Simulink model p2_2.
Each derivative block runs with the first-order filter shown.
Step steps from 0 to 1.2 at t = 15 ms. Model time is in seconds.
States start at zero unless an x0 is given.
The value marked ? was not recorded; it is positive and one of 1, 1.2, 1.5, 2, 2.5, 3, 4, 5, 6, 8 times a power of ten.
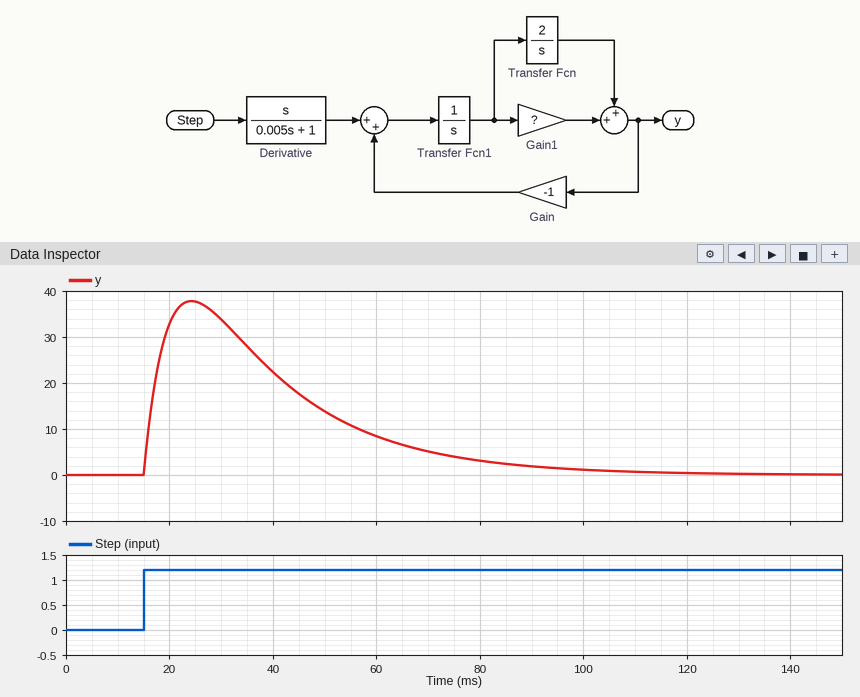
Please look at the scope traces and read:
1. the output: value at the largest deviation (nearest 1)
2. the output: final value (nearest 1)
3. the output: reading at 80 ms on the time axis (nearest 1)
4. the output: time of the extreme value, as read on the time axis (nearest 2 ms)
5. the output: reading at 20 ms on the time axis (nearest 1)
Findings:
38
0
3
24 ms
33
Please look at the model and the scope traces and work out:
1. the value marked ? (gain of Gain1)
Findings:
50
